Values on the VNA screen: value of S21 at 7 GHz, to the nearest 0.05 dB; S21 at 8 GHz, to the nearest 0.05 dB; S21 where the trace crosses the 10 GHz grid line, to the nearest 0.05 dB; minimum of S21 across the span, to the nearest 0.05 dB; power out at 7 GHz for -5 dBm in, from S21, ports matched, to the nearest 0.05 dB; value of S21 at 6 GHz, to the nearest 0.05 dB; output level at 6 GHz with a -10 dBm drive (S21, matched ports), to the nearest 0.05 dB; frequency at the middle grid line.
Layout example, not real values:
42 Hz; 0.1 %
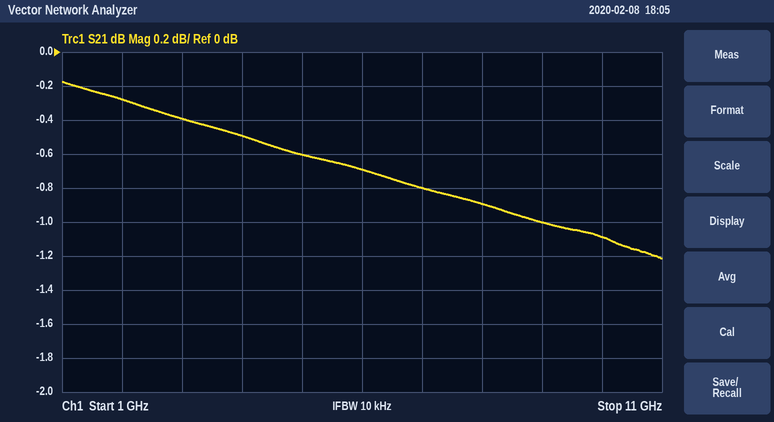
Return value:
-0.80 dB; -0.90 dB; -1.10 dB; -1.20 dB; -5.80 dBm; -0.70 dB; -10.70 dBm; 6 GHz
